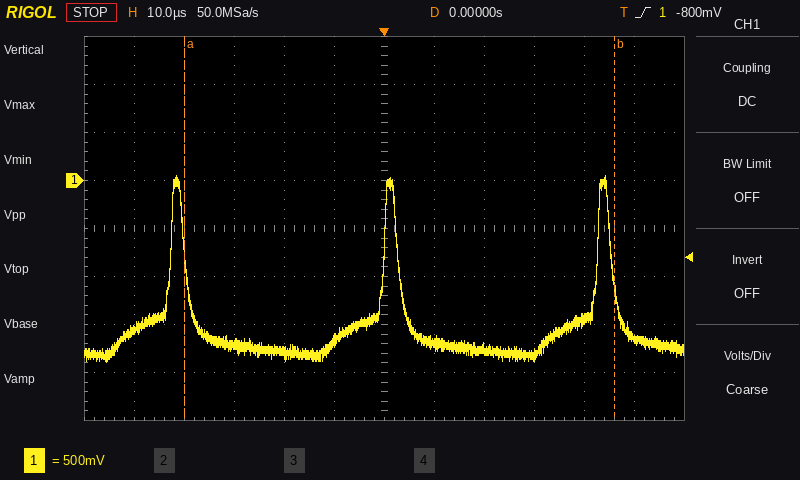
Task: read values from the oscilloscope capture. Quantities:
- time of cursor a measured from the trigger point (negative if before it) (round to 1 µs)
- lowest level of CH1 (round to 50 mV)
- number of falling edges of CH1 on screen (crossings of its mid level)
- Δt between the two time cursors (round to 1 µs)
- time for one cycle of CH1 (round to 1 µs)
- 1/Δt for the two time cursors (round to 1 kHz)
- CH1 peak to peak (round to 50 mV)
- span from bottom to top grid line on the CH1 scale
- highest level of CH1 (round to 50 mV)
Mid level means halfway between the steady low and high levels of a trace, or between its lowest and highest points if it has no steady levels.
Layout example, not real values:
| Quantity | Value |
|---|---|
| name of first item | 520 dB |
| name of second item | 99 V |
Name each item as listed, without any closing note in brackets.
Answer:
| Quantity | Value |
|---|---|
| time of cursor a measured from the trigger point (negative if before it) | -40 µs |
| lowest level of CH1 | -1.90 V |
| number of falling edges of CH1 on screen | 3 |
| Δt between the two time cursors | 86 µs |
| time for one cycle of CH1 | 43 µs |
| 1/Δt for the two time cursors | 12 kHz |
| CH1 peak to peak | 1.95 V |
| span from bottom to top grid line on the CH1 scale | 4 V |
| highest level of CH1 | 50 mV |
